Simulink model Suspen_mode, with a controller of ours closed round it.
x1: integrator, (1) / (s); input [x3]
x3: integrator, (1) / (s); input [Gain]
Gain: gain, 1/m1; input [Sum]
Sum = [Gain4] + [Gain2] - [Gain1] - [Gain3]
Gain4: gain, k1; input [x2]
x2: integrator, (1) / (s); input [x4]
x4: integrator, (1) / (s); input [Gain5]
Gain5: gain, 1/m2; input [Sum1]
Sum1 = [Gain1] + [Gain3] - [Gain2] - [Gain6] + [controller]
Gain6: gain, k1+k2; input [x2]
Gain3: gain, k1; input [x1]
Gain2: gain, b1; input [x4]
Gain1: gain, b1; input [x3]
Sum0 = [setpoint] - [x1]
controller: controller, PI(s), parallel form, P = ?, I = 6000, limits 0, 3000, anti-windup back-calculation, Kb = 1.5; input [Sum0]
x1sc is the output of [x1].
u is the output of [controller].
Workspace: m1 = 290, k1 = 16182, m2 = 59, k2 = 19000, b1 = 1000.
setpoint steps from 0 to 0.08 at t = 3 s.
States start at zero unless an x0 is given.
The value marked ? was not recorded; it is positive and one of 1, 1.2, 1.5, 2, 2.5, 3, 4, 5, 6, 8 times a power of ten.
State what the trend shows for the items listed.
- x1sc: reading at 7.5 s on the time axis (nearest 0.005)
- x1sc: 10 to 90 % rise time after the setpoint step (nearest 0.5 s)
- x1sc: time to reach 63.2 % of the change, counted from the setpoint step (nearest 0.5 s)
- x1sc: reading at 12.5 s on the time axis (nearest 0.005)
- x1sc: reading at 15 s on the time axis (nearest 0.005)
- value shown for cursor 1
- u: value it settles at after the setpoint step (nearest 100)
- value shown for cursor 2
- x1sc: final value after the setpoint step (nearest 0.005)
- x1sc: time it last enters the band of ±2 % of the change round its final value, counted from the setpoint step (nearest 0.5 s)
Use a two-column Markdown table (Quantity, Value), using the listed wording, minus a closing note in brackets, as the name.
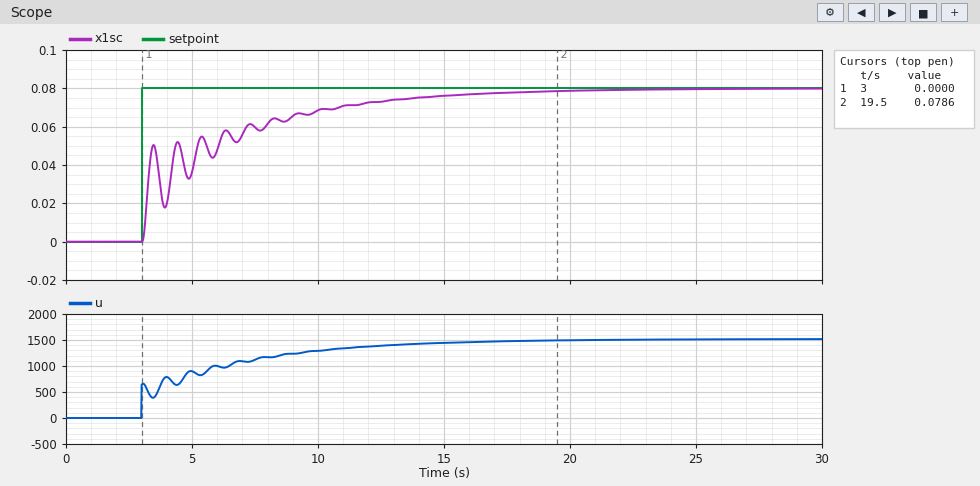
| Quantity | Value |
|---|---|
| x1sc: reading at 7.5 s on the time axis | 0.060 |
| x1sc: 10 to 90 % rise time after the setpoint step | 8.5 s |
| x1sc: time to reach 63.2 % of the change, counted from the setpoint step | 1.5 s |
| x1sc: reading at 12.5 s on the time axis | 0.075 |
| x1sc: reading at 15 s on the time axis | 0.075 |
| value shown for cursor 1 | 0.0000 |
| u: value it settles at after the setpoint step | 1500 |
| value shown for cursor 2 | 0.0786 |
| x1sc: final value after the setpoint step | 0.080 |
| x1sc: time it last enters the band of ±2 % of the change round its final value, counted from the setpoint step | 16.0 s |
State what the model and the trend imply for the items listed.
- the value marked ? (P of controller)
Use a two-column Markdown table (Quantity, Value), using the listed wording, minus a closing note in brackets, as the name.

| Quantity | Value |
|---|---|
| the value marked ? | 8000 |
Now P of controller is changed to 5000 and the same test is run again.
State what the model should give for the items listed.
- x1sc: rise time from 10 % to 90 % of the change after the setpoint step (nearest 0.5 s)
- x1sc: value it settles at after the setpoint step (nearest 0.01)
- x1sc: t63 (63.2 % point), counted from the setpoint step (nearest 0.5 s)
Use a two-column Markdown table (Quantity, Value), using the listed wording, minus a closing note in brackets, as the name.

| Quantity | Value |
|---|---|
| x1sc: rise time from 10 % to 90 % of the change after the setpoint step | 8.0 s |
| x1sc: value it settles at after the setpoint step | 0.08 |
| x1sc: t63 (63.2 % point), counted from the setpoint step | 2.5 s |
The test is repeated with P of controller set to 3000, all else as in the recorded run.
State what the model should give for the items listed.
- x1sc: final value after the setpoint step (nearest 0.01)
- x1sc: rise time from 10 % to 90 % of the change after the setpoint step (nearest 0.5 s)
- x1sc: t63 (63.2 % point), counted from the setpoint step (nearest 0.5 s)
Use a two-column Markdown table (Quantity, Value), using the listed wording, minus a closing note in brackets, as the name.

| Quantity | Value |
|---|---|
| x1sc: final value after the setpoint step | 0.08 |
| x1sc: rise time from 10 % to 90 % of the change after the setpoint step | 7.5 s |
| x1sc: t63 (63.2 % point), counted from the setpoint step | 2.5 s |
